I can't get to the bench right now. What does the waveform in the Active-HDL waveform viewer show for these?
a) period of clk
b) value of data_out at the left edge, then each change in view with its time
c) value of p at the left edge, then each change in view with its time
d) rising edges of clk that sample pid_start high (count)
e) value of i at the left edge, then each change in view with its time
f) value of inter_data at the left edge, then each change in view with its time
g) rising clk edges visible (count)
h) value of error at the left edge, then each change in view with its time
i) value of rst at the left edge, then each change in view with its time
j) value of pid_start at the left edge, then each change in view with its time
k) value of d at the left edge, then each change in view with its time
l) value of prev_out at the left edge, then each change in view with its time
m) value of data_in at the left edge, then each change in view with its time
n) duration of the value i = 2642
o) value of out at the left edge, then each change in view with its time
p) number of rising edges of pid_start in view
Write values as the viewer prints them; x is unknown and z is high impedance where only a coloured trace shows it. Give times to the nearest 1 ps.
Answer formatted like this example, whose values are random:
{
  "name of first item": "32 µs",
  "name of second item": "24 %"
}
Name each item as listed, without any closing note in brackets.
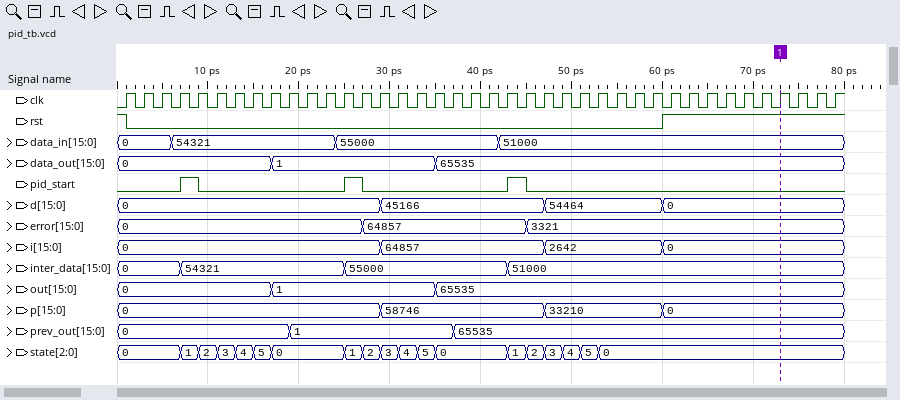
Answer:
{
  "period of clk": "2 ps",
  "value of data_out at the left edge, then each change in view with its time": "0, 1 at 17 ps, 65535 at 35 ps",
  "value of p at the left edge, then each change in view with its time": "0, 58746 at 29 ps, 33210 at 47 ps, 0 at 60 ps",
  "rising edges of clk that sample pid_start high": "3",
  "value of i at the left edge, then each change in view with its time": "0, 64857 at 29 ps, 2642 at 47 ps, 0 at 60 ps",
  "value of inter_data at the left edge, then each change in view with its time": "0, 54321 at 7 ps, 55000 at 25 ps, 51000 at 43 ps",
  "rising clk edges visible": "40",
  "value of error at the left edge, then each change in view with its time": "0, 64857 at 27 ps, 3321 at 45 ps",
  "value of rst at the left edge, then each change in view with its time": "1, 0 at 1 ps, 1 at 60 ps",
  "value of pid_start at the left edge, then each change in view with its time": "0, 1 at 7 ps, 0 at 9 ps, 1 at 25 ps, 0 at 27 ps, 1 at 43 ps, 0 at 45 ps",
  "value of d at the left edge, then each change in view with its time": "0, 45166 at 29 ps, 54464 at 47 ps, 0 at 60 ps",
  "value of prev_out at the left edge, then each change in view with its time": "0, 1 at 19 ps, 65535 at 37 ps",
  "value of data_in at the left edge, then each change in view with its time": "0, 54321 at 6 ps, 55000 at 24 ps, 51000 at 42 ps",
  "duration of the value i = 2642": "13 ps",
  "value of out at the left edge, then each change in view with its time": "0, 1 at 17 ps, 65535 at 35 ps",
  "number of rising edges of pid_start in view": "3"
}
